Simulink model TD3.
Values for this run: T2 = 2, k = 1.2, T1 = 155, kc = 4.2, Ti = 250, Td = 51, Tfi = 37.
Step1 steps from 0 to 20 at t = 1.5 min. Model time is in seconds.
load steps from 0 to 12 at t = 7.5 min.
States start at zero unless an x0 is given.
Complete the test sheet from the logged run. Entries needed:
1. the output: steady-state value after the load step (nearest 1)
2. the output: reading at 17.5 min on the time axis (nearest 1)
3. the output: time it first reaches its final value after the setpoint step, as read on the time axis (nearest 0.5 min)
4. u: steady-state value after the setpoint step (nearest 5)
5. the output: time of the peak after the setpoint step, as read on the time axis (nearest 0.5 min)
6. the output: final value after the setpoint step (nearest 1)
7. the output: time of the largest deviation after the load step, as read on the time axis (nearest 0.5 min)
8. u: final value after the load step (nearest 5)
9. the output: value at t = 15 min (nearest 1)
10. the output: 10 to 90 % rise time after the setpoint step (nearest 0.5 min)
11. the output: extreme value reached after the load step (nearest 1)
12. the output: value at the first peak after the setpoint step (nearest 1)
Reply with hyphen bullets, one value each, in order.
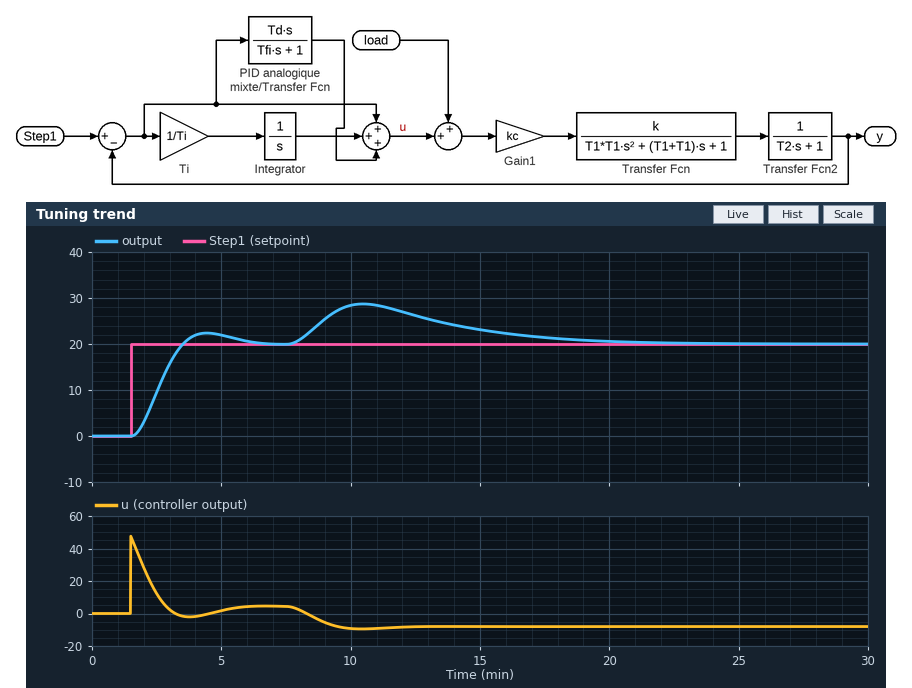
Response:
- 20
- 21
- 3.5 min
- 5
- 4.5 min
- 20
- 10.5 min
- -10
- 23
- 1.5 min
- 29
- 22
